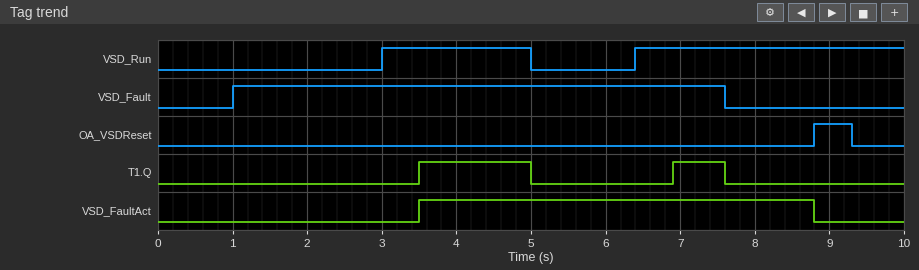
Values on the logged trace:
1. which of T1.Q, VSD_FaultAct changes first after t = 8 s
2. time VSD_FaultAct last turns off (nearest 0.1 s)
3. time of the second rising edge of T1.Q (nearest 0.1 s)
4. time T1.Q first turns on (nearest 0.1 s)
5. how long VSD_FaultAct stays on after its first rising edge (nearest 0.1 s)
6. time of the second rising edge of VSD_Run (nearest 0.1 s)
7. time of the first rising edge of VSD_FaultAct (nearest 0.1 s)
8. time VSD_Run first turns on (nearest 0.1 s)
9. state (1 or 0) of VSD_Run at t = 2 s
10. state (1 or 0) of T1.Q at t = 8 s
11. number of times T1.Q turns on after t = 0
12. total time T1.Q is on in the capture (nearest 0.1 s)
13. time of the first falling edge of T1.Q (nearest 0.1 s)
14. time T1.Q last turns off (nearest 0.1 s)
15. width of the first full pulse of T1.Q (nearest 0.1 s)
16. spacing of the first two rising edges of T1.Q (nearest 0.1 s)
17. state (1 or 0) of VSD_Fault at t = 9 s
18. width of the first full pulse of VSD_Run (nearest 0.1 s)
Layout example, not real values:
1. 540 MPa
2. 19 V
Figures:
1. VSD_FaultAct
2. 8.8 s
3. 6.9 s
4. 3.5 s
5. 5.3 s
6. 6.4 s
7. 3.5 s
8. 3.0 s
9. 0
10. 0
11. 2
12. 2.2 s
13. 5.0 s
14. 7.6 s
15. 1.5 s
16. 3.4 s
17. 0
18. 2.0 s
